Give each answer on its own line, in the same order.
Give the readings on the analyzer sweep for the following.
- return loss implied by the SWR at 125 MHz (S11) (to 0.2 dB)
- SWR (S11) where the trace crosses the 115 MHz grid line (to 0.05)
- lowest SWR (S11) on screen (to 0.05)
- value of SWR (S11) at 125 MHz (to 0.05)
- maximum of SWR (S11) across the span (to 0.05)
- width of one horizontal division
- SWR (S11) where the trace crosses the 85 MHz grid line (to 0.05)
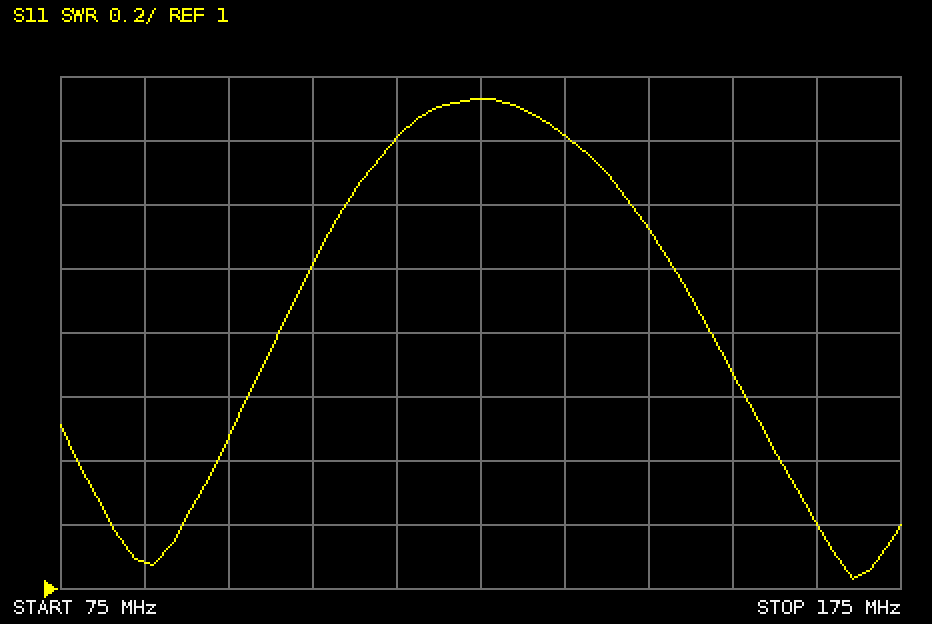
7.2 dB
2.40
1.05
2.55
2.55
10 MHz
1.10
